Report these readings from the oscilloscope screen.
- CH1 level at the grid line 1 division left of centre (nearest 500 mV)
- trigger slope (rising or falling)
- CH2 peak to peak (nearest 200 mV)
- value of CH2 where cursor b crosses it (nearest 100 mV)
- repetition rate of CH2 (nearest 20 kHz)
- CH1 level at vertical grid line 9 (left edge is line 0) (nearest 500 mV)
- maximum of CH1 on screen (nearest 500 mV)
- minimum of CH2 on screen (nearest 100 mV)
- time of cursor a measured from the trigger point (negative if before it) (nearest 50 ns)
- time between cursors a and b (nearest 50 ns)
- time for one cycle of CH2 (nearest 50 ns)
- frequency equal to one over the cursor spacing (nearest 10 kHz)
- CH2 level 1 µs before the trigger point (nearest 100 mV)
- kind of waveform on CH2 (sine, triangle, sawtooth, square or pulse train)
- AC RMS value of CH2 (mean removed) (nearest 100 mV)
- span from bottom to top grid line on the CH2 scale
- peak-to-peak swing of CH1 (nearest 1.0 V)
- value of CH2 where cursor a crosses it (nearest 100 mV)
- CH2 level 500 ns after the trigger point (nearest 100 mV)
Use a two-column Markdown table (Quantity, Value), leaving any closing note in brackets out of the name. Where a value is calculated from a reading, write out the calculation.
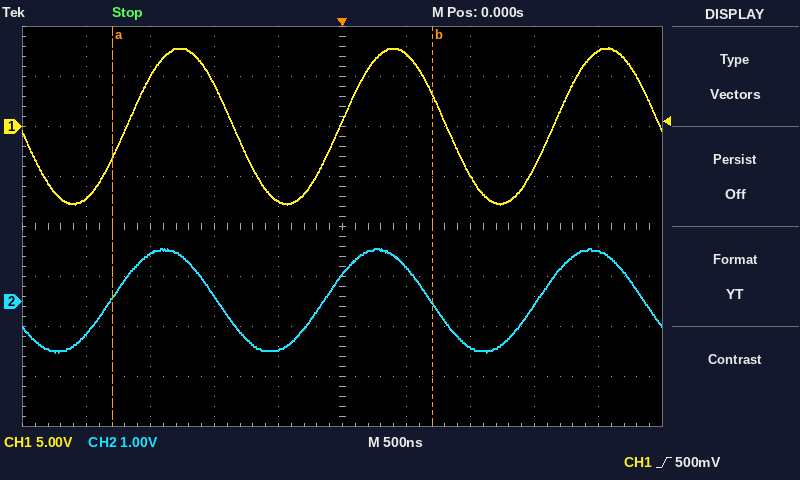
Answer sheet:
| Quantity | Value |
|---|---|
| CH1 level at the grid line 1 division left of centre | -7.5 V |
| trigger slope | rising |
| CH2 peak to peak | 2.0 V |
| value of CH2 where cursor b crosses it | 0.0 V |
| repetition rate of CH2 | 1 / 1.65 µs ≈ 606 kHz, so 600 kHz to the nearest 20 kHz |
| CH1 level at vertical grid line 9 (left edge is line 0) | 7.5 V |
| maximum of CH1 on screen | 8.0 V |
| minimum of CH2 on screen | -1.0 V |
| time of cursor a measured from the trigger point (negative if before it) | -1.80 µs |
| time between cursors a and b | 2.50 µs |
| time for one cycle of CH2 | 1.65 µs |
| frequency equal to one over the cursor spacing | 1 / 2.50 µs ≈ 400 kHz |
| CH2 level 1 µs before the trigger point | 100 mV |
| kind of waveform on CH2 | sine |
| AC RMS value of CH2 (mean removed) | 2.0 V / (2√2) ≈ 707 mV, so 700 mV to the nearest 100 mV |
| span from bottom to top grid line on the CH2 scale | 8 V |
| peak-to-peak swing of CH1 | 16.0 V |
| value of CH2 where cursor a crosses it | 100 mV |
| CH2 level 500 ns after the trigger point | 700 mV |
